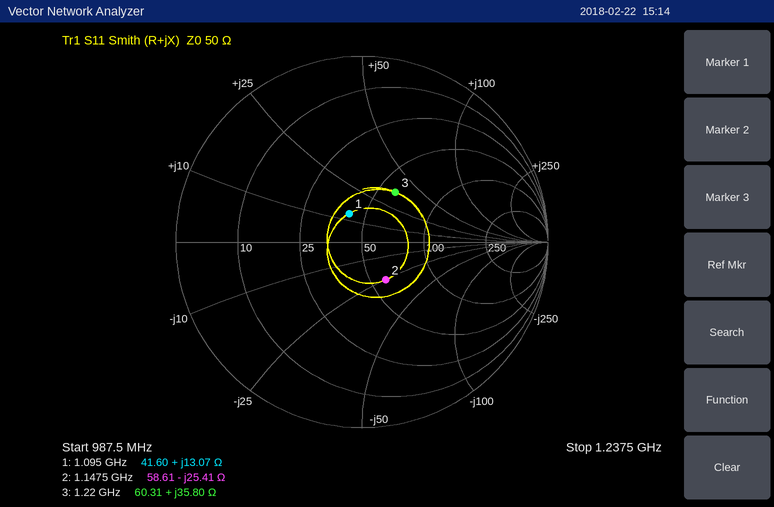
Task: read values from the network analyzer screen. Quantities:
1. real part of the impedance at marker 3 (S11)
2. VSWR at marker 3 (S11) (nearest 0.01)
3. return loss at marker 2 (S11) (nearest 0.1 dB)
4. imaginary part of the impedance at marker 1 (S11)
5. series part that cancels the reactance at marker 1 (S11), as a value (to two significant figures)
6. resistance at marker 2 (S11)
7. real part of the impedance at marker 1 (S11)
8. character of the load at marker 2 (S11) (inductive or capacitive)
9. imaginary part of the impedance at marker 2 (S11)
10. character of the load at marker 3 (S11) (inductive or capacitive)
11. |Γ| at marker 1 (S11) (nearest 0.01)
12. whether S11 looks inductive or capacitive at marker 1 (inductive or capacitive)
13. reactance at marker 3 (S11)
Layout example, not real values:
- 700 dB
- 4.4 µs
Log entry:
- 60.31 Ω
- 1.95
- 12.4 dB
- +13.07 Ω
- 11 pF
- 58.61 Ω
- 41.60 Ω
- capacitive
- -25.41 Ω
- inductive
- 0.17
- inductive
- +35.80 Ω
